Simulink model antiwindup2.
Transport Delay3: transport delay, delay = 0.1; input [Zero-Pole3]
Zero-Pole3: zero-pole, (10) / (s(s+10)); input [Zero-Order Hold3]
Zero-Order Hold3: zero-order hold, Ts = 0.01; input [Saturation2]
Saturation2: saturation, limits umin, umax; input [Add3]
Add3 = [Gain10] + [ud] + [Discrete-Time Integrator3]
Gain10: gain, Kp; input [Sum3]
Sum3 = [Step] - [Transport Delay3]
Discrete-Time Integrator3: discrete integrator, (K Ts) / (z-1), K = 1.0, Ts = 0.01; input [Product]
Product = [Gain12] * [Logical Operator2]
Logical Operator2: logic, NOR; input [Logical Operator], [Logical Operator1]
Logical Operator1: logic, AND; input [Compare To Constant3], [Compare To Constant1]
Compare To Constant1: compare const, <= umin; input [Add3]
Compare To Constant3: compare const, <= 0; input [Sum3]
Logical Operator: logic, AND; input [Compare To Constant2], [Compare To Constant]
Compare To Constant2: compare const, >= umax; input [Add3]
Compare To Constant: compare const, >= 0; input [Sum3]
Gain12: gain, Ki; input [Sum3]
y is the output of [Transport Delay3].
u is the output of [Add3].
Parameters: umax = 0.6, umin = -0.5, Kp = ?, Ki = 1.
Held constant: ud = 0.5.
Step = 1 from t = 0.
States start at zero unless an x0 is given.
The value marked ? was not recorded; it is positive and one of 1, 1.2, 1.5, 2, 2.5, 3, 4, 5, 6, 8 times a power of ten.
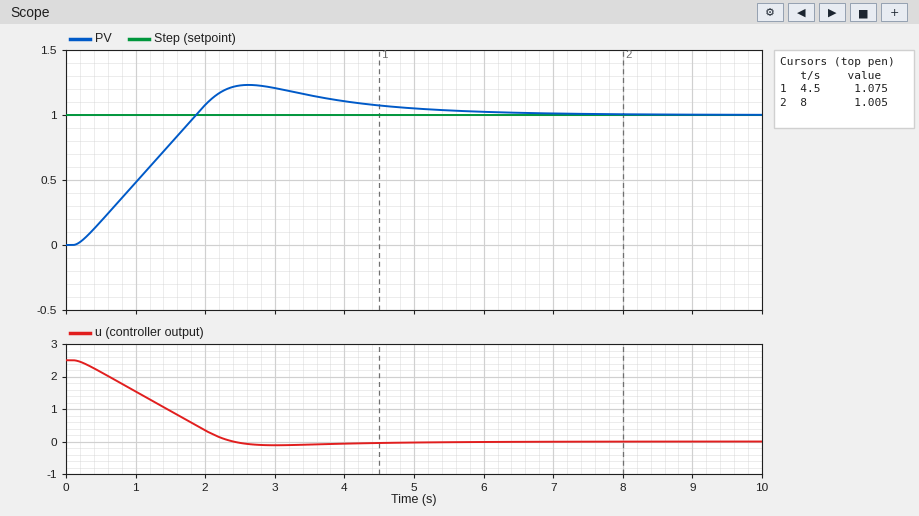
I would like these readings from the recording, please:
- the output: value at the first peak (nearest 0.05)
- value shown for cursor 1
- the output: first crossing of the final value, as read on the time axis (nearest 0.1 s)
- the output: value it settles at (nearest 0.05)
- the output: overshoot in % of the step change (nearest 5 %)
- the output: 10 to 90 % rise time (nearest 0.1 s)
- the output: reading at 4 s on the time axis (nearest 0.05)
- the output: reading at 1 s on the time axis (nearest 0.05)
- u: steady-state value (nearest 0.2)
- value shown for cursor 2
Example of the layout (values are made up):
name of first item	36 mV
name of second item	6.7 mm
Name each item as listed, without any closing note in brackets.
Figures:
the output: value at the first peak	1.25
value shown for cursor 1	1.075
the output: first crossing of the final value, as read on the time axis	1.9 s
the output: value it settles at	1.00
the output: overshoot in % of the step change	25 %
the output: 10 to 90 % rise time	1.3 s
the output: reading at 4 s on the time axis	1.10
the output: reading at 1 s on the time axis	0.50
u: steady-state value	0.0
value shown for cursor 2	1.005
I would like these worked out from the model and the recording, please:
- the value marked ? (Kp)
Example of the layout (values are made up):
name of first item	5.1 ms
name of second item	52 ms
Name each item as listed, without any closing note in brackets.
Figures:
the value marked ?	2
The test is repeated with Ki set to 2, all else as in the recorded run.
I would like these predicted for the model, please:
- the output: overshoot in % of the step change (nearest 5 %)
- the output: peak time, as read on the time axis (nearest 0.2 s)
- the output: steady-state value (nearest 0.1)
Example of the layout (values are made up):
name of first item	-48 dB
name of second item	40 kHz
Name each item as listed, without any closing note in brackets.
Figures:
the output: overshoot in % of the step change	20 %
the output: peak time, as read on the time axis	2.6 s
the output: steady-state value	1.0
